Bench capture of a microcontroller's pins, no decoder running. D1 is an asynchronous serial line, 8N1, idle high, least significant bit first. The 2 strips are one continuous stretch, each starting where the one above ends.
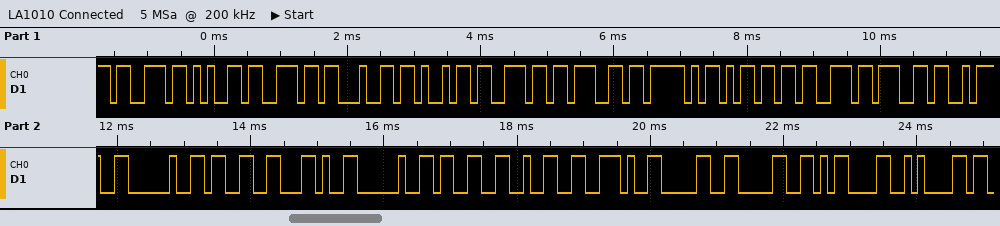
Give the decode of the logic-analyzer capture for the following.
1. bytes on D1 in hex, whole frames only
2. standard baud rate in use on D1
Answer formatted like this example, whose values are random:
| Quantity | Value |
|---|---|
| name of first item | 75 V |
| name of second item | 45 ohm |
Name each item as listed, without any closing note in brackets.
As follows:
| Quantity | Value |
|---|---|
| bytes on D1 in hex, whole frames only | 73 65 6E 64 69 6E 67 5F 6D 73 67 3A 20 33 2C 20 33 32 2E 30 30 0D 0A |
| standard baud rate in use on D1 | 9600 baud |
